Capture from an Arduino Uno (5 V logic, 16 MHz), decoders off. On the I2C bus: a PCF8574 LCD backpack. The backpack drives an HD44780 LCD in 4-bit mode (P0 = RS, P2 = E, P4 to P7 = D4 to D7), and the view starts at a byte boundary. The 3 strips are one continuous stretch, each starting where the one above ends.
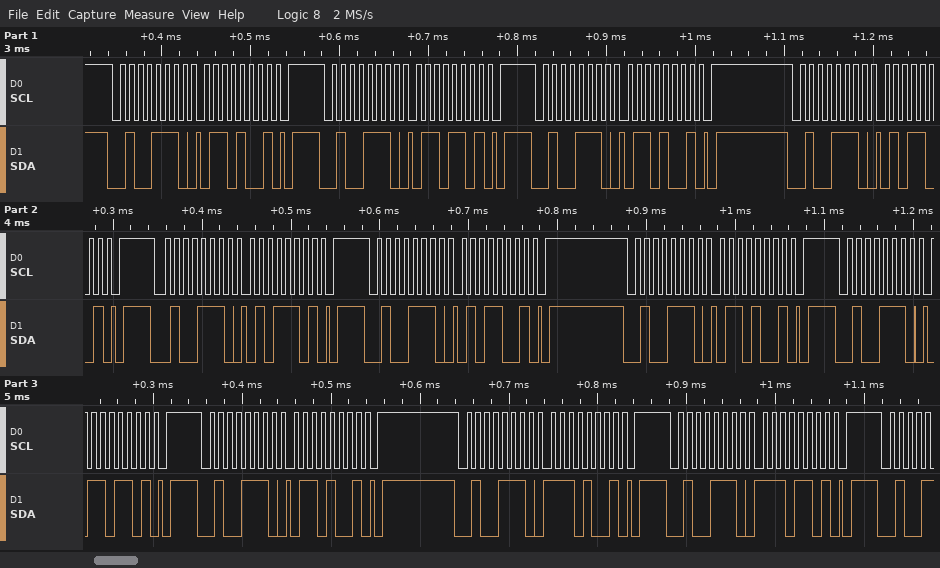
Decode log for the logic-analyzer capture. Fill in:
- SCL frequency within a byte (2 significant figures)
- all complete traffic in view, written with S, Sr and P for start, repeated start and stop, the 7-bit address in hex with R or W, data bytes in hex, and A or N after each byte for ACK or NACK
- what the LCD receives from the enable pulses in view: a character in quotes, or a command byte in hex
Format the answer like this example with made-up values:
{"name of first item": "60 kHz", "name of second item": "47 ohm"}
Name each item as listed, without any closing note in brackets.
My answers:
{"SCL frequency within a byte": "100 kHz", "all complete traffic in view, written with S, Sr and P for start, repeated start and stop, the 7-bit address in hex with R or W, data bytes in hex, and A or N after each byte for ACK or NACK": "S 27W A 69 A P S 27W A 6D A P S 27W A 69 A P S 27W A 59 A P S 27W A 5D A P S 27W A 59 A P S 27W A 69 A P S 27W A 6D A P S 27W A 69 A P S 27W A E9 A P S 27W A ED A P", "what the LCD receives from the enable pulses in view: a character in quotes, or a command byte in hex": "'e'"}
